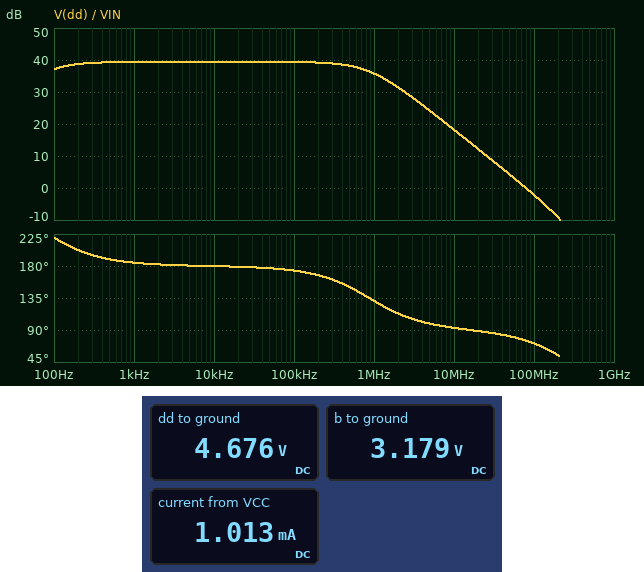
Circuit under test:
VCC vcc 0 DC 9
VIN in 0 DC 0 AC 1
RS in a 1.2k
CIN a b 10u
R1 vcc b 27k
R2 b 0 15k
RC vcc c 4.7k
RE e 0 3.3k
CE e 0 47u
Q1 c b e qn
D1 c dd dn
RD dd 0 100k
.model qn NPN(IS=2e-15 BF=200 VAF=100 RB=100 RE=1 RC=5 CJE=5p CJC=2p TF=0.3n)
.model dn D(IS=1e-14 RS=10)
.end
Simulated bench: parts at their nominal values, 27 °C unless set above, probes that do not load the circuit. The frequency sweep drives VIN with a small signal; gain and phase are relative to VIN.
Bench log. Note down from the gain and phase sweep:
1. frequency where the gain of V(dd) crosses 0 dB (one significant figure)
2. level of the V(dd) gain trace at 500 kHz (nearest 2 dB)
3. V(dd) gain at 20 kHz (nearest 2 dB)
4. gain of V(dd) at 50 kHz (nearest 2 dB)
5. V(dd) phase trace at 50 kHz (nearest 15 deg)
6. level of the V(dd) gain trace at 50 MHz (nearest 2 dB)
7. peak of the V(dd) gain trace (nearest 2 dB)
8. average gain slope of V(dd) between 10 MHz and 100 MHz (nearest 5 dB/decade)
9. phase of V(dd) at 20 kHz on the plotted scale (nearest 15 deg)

80 MHz
38 dB
40 dB
40 dB
180 deg
4 dB
40 dB
-20 dB/decade
180 deg
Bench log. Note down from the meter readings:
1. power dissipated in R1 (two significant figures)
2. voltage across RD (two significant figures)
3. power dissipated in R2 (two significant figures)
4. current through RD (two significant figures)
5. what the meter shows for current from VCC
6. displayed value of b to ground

1.3 mW
4.7 V
670 µW
47 µA
1.013 mA
3.179 V
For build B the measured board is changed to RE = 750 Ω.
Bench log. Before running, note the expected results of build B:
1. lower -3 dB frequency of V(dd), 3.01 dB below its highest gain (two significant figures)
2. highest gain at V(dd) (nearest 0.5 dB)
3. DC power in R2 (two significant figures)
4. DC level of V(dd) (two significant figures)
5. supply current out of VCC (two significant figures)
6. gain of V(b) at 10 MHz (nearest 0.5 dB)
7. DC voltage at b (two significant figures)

6.8 Hz
-17.0 dB
270 µW
850 mV
1.9 mA
-20.5 dB
2.0 V
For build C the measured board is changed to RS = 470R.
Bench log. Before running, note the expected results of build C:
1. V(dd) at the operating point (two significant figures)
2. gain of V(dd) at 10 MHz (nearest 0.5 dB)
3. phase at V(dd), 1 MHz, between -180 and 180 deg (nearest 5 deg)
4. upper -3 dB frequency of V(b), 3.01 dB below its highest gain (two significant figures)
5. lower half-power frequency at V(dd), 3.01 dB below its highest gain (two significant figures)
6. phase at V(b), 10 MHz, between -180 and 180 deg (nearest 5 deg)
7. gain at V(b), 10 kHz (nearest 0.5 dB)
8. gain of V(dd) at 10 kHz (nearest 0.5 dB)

4.7 V
25.0 dB
150 deg
1.7 MHz
89 Hz
-25 deg
-1.0 dB
40.5 dB
